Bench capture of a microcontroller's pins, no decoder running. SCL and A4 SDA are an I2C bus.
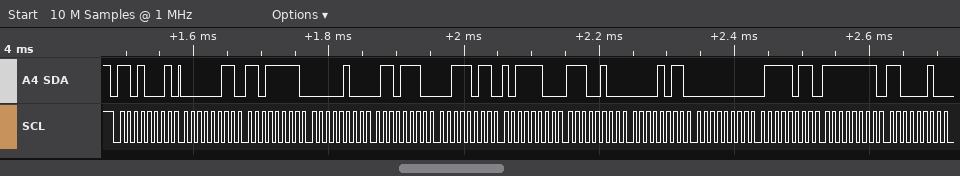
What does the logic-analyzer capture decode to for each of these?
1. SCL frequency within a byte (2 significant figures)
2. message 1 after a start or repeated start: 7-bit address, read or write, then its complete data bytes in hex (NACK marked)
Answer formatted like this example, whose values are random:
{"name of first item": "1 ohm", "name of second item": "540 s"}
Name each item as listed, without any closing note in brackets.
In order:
{"SCL frequency within a byte": "100 kHz", "message 1 after a start or repeated start: 7-bit address, read or write, then its complete data bytes in hex": "0x68 read: 03 DF 04 6E 3B BC E4 0B 00 7B FF C2"}
